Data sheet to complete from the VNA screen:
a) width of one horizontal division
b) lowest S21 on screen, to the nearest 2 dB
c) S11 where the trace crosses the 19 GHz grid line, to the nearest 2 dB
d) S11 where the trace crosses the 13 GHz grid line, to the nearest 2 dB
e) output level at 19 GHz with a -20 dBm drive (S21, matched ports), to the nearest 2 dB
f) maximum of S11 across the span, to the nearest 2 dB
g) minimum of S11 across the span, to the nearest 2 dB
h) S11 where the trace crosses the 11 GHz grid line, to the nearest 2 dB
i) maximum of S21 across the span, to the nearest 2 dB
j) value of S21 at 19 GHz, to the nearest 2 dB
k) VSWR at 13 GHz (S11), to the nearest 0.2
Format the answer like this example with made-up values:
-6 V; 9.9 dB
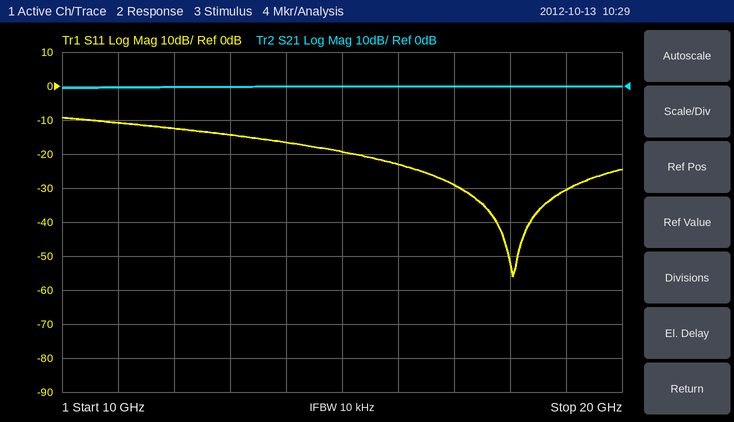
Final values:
1 GHz; 0 dB; -30 dB; -14 dB; -20 dBm; -10 dB; -56 dB; -10 dB; 0 dB; 0 dB; 1.4
